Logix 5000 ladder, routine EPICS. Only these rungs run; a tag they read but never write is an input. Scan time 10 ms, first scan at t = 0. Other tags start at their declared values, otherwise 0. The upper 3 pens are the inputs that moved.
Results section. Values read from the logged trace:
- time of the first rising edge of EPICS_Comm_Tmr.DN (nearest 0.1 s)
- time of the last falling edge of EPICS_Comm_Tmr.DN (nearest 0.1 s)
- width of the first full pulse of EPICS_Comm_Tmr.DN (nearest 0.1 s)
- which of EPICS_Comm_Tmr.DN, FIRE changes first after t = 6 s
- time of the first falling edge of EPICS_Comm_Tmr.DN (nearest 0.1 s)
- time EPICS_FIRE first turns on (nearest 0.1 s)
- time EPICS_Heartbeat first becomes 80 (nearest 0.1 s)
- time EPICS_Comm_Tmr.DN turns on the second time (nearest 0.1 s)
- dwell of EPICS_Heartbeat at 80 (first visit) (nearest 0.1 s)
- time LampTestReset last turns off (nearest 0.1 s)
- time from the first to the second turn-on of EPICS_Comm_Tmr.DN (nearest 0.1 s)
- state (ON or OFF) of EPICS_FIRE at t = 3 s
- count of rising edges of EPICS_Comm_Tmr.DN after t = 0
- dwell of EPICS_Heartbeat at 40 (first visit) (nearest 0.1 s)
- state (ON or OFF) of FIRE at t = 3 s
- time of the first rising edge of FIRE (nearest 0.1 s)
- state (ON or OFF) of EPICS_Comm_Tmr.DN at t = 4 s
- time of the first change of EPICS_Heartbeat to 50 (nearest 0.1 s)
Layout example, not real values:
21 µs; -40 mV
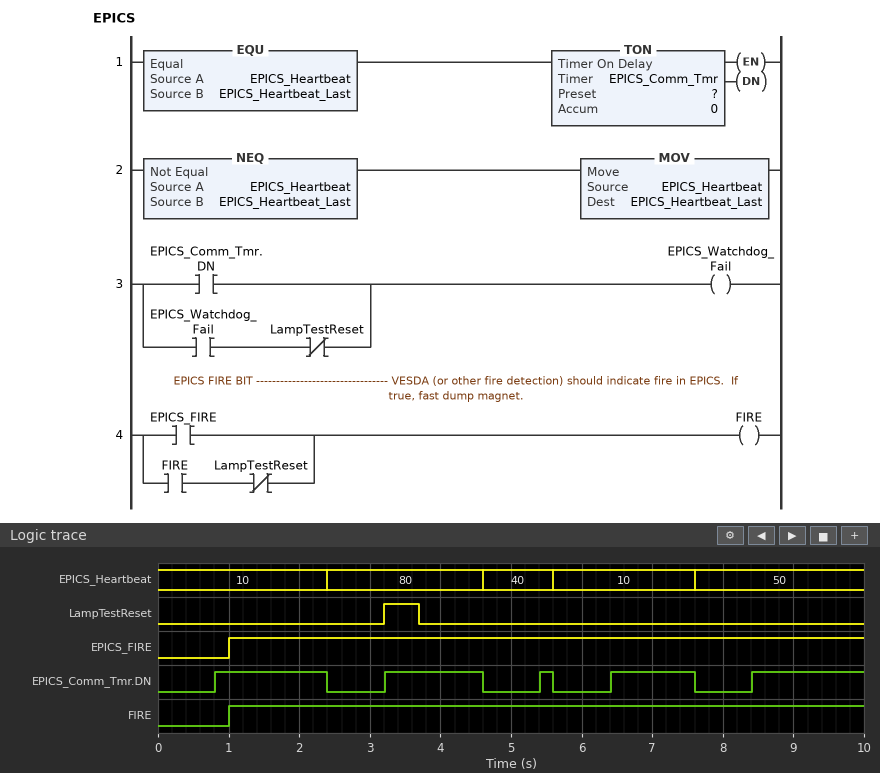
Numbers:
0.8 s; 7.6 s; 1.6 s; EPICS_Comm_Tmr.DN; 2.4 s; 1.0 s; 2.4 s; 3.2 s; 2.2 s; 3.7 s; 2.4 s; ON; 5; 1.0 s; ON; 1.0 s; ON; 7.6 s
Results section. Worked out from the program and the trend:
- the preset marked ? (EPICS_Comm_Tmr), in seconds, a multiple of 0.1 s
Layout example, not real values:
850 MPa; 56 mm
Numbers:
0.8 s
